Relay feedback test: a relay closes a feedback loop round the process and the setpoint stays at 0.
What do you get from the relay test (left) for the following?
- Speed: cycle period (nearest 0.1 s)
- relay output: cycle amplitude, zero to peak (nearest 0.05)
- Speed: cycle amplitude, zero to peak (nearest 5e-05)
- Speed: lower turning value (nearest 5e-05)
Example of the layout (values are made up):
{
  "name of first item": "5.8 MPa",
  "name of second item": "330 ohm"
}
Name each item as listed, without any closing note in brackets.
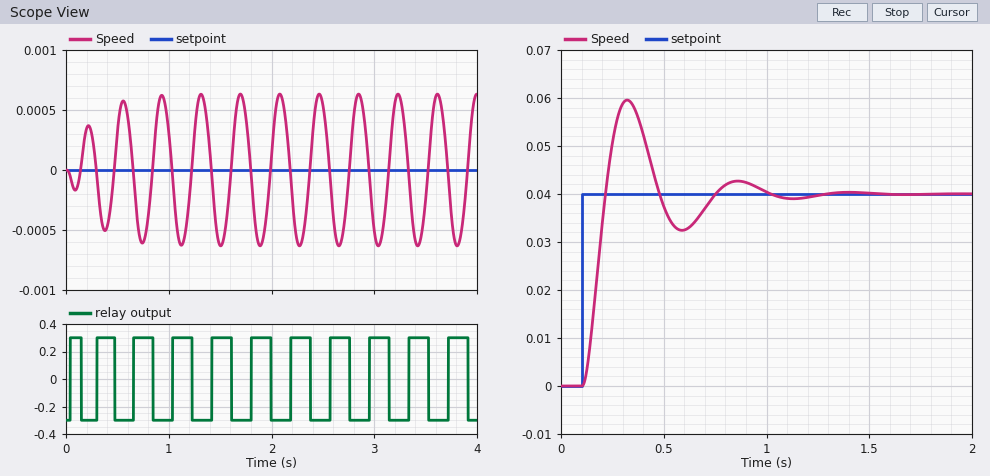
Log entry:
{
  "Speed: cycle period": "0.4 s",
  "relay output: cycle amplitude, zero to peak": "0.30",
  "Speed: cycle amplitude, zero to peak": "0.00065",
  "Speed: lower turning value": "-0.00065"
}
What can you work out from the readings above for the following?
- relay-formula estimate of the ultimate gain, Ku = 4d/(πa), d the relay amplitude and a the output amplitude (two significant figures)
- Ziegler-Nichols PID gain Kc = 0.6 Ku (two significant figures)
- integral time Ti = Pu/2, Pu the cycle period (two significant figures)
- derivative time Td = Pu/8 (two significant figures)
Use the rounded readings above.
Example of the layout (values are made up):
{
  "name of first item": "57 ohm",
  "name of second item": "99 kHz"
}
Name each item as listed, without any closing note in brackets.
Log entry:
{
  "relay-formula estimate of the ultimate gain, Ku = 4d/(πa), d the relay amplitude and a the output amplitude": "590",
  "Ziegler-Nichols PID gain Kc = 0.6 Ku": "350",
  "integral time Ti = Pu/2, Pu the cycle period": "0.20 s",
  "derivative time Td = Pu/8": "0.050 s"
}
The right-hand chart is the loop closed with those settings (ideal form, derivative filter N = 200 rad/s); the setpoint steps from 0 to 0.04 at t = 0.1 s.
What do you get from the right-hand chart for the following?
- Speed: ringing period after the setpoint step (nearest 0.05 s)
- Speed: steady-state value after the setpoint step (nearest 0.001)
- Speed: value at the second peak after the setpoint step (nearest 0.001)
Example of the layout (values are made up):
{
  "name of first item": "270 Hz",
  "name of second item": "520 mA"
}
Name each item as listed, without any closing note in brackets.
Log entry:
{
  "Speed: ringing period after the setpoint step": "0.55 s",
  "Speed: steady-state value after the setpoint step": "0.040",
  "Speed: value at the second peak after the setpoint step": "0.043"
}
